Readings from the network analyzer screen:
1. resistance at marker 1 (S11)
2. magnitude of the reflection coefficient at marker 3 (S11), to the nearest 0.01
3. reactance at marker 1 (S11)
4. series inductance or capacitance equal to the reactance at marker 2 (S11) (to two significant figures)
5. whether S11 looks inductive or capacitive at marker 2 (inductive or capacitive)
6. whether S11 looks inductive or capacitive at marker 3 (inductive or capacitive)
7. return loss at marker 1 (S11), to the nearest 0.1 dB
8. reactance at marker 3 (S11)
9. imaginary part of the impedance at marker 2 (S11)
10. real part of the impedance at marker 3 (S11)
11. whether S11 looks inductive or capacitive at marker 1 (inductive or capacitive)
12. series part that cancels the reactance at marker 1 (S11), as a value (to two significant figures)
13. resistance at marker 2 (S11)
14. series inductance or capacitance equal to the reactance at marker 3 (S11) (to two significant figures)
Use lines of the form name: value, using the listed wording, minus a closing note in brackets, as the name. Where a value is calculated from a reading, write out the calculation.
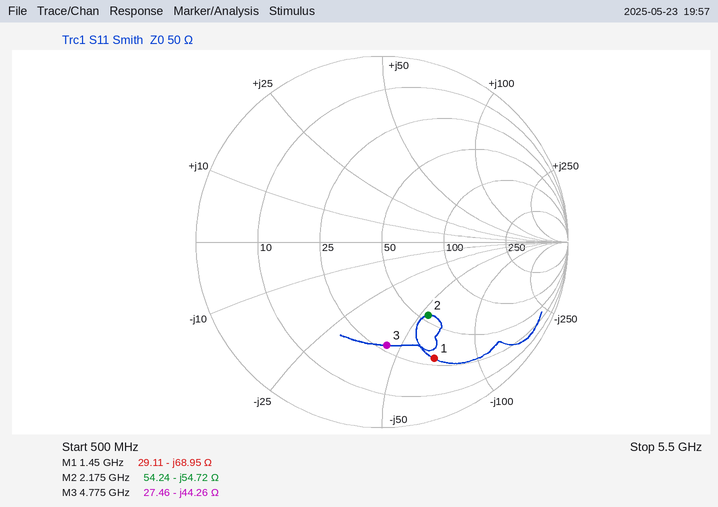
resistance at marker 1: 29.11 Ω
magnitude of the reflection coefficient at marker 3 (S11), to the nearest 0.01: 0.56
reactance at marker 1: -68.95 Ω
series inductance or capacitance equal to the reactance at marker 2 (S11): C = 1/(2π × 2.175 GHz × 54.72 Ω) ≈ 1.3 pF
whether S11 looks inductive or capacitive at marker 2: capacitive
whether S11 looks inductive or capacitive at marker 3: capacitive
return loss at marker 1 (S11), to the nearest 0.1 dB: 3.3 dB
reactance at marker 3: -44.26 Ω
imaginary part of the impedance at marker 2: -54.72 Ω
real part of the impedance at marker 3: 27.46 Ω
whether S11 looks inductive or capacitive at marker 1: capacitive
series part that cancels the reactance at marker 1 (S11), as a value: L = 68.95 Ω/(2π × 1.45 GHz) ≈ 7.6 nH
resistance at marker 2: 54.24 Ω
series inductance or capacitance equal to the reactance at marker 3 (S11): C = 1/(2π × 4.775 GHz × 44.26 Ω) ≈ 753 fF, so 750 fF to two significant figures
